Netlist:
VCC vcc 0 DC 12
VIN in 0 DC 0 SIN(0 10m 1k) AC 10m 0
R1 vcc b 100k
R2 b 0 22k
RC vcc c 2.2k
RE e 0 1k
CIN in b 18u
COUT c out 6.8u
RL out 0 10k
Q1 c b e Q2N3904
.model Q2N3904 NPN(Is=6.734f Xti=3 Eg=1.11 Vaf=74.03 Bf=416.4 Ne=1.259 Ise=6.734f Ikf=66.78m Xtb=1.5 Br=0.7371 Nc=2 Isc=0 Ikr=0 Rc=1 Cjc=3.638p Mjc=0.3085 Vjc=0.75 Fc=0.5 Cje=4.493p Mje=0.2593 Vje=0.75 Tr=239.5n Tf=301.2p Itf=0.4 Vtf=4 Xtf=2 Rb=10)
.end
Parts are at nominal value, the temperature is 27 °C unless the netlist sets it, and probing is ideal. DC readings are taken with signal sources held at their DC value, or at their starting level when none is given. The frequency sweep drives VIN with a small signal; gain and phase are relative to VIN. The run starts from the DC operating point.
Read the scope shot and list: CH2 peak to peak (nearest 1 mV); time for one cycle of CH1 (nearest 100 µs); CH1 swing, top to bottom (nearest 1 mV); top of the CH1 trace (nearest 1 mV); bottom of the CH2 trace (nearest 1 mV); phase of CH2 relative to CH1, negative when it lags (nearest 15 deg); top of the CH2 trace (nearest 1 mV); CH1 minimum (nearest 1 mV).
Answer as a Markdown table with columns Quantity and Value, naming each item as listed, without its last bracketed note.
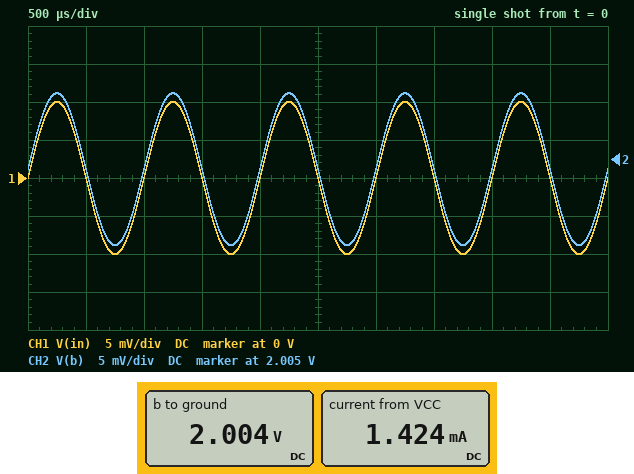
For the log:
| Quantity | Value |
|---|---|
| CH2 peak to peak | 20 mV |
| time for one cycle of CH1 | 1.0 ms |
| CH1 swing, top to bottom | 20 mV |
| top of the CH1 trace | 10 mV |
| bottom of the CH2 trace | 1.994 V |
| phase of CH2 relative to CH1, negative when it lags | 0 deg |
| top of the CH2 trace | 2.014 V |
| CH1 minimum | -10 mV |
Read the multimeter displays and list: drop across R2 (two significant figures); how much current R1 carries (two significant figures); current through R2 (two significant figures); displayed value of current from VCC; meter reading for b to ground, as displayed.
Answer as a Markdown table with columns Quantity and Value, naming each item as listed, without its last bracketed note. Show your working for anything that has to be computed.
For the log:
| Quantity | Value |
|---|---|
| drop across R2 | 2.004 V = 2.0 V |
| how much current R1 carries | (12 V - 2.004 V) / 100 kΩ = 100 µA |
| current through R2 | (2.004 V) / 22 kΩ = 91 µA |
| displayed value of current from VCC | 1.424 mA |
| meter reading for b to ground, as displayed | 2.004 V |
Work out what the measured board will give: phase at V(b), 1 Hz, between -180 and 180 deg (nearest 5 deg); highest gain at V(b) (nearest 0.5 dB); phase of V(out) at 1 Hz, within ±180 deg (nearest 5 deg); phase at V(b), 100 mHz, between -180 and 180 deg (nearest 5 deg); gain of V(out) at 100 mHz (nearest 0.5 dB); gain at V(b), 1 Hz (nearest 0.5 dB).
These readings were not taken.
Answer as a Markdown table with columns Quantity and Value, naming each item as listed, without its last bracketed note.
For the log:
| Quantity | Value |
|---|---|
| phase at V(b), 1 Hz, between -180 and 180 deg | 30 deg |
| highest gain at V(b) | 0 dB |
| phase of V(out) at 1 Hz, within ±180 deg | -90 deg |
| phase at V(b), 100 mHz, between -180 and 180 deg | 80 deg |
| gain of V(out) at 100 mHz | -35.5 dB |
| gain at V(b), 1 Hz | -1.0 dB |
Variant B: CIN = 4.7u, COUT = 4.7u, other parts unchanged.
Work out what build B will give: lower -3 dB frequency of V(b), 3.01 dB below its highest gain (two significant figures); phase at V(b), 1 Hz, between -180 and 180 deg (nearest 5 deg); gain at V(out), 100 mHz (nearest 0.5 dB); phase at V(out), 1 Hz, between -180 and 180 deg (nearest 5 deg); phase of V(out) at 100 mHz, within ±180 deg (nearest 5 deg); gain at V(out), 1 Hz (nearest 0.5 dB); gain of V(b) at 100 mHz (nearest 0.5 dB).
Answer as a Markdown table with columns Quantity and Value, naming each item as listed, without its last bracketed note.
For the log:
| Quantity | Value |
|---|---|
| lower -3 dB frequency of V(b), 3.01 dB below its highest gain | 2.1 Hz |
| phase at V(b), 1 Hz, between -180 and 180 deg | 65 deg |
| gain at V(out), 100 mHz | -50.5 dB |
| phase at V(out), 1 Hz, between -180 and 180 deg | -45 deg |
| phase of V(out) at 100 mHz, within ±180 deg | -5 deg |
| gain at V(out), 1 Hz | -12.0 dB |
| gain of V(b) at 100 mHz | -26.5 dB |
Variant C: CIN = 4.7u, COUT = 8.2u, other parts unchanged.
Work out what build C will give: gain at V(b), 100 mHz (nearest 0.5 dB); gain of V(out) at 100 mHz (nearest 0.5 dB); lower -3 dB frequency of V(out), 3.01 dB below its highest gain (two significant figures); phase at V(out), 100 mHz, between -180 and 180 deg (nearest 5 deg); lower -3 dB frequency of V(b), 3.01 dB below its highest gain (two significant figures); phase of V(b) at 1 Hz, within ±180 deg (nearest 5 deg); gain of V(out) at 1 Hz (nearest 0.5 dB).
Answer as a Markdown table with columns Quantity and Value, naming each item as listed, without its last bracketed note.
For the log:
| Quantity | Value |
|---|---|
| gain at V(b), 100 mHz | -26.5 dB |
| gain of V(out) at 100 mHz | -45.5 dB |
| lower -3 dB frequency of V(out), 3.01 dB below its highest gain | 2.9 Hz |
| phase at V(out), 100 mHz, between -180 and 180 deg | -5 deg |
| lower -3 dB frequency of V(b), 3.01 dB below its highest gain | 2.1 Hz |
| phase of V(b) at 1 Hz, within ±180 deg | 65 deg |
| gain of V(out) at 1 Hz | -8.0 dB |
